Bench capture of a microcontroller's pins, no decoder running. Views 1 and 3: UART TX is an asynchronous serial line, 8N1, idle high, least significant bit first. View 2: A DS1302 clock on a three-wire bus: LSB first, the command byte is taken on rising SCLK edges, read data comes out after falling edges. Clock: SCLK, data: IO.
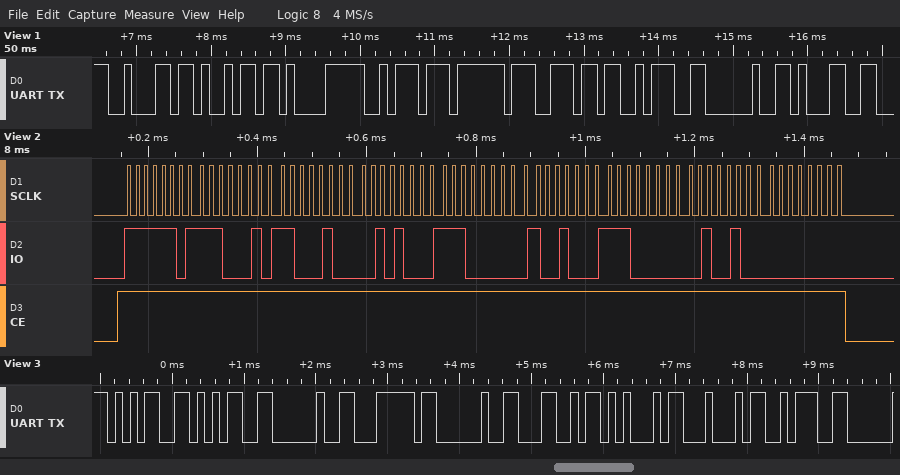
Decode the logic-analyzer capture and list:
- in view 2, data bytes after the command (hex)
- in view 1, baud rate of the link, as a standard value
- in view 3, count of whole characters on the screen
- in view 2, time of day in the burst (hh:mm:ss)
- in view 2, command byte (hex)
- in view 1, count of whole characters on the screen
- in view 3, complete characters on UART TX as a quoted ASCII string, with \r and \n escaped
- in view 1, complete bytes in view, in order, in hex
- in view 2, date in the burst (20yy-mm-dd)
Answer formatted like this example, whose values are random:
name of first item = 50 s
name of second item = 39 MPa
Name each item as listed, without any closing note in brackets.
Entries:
in view 2, data bytes after the command = 47 23 14 07 12 07 24 00
in view 1, baud rate of the link, as a standard value = 9600 baud
in view 3, count of whole characters on the screen = 9
in view 2, time of day in the burst = 14:23:47
in view 2, command byte = 0xBF
in view 1, count of whole characters on the screen = 9
in view 3, complete characters on UART TX as a quoted ASCII string, with \r and \n escaped = "55 | LED:"
in view 1, complete bytes in view, in order, in hex = 62 69 E1 BA BF 6E 3A 20 31
in view 2, date in the burst = 2024-12-07
